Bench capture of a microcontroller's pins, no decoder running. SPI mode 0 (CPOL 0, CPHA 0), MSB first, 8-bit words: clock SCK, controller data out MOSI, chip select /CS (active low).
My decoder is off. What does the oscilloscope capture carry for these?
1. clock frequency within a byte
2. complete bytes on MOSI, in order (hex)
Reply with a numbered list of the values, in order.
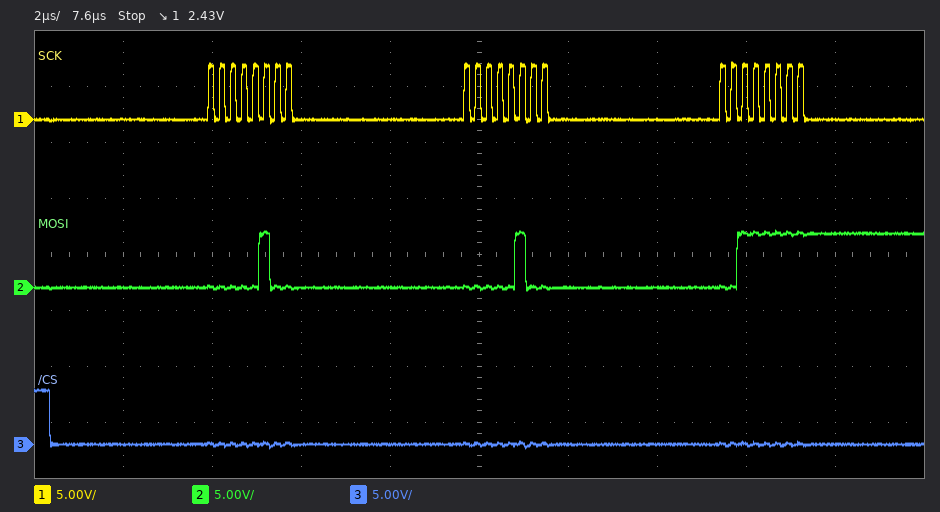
1. 4 MHz
2. 04 04 3F
